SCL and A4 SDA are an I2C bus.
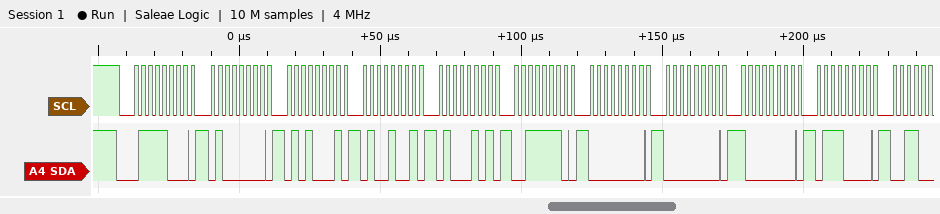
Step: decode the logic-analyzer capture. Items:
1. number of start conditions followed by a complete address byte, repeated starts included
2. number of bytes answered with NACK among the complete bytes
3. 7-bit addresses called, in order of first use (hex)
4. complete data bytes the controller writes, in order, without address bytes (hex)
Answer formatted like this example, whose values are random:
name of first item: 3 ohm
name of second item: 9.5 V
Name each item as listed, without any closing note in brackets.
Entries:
number of start conditions followed by a complete address byte, repeated starts included: 1
number of bytes answered with NACK among the complete bytes: 0
7-bit addresses called, in order of first use: 0x3C
complete data bytes the controller writes, in order, without address bytes: 40 51 49 45 3E 00 00 80 70
